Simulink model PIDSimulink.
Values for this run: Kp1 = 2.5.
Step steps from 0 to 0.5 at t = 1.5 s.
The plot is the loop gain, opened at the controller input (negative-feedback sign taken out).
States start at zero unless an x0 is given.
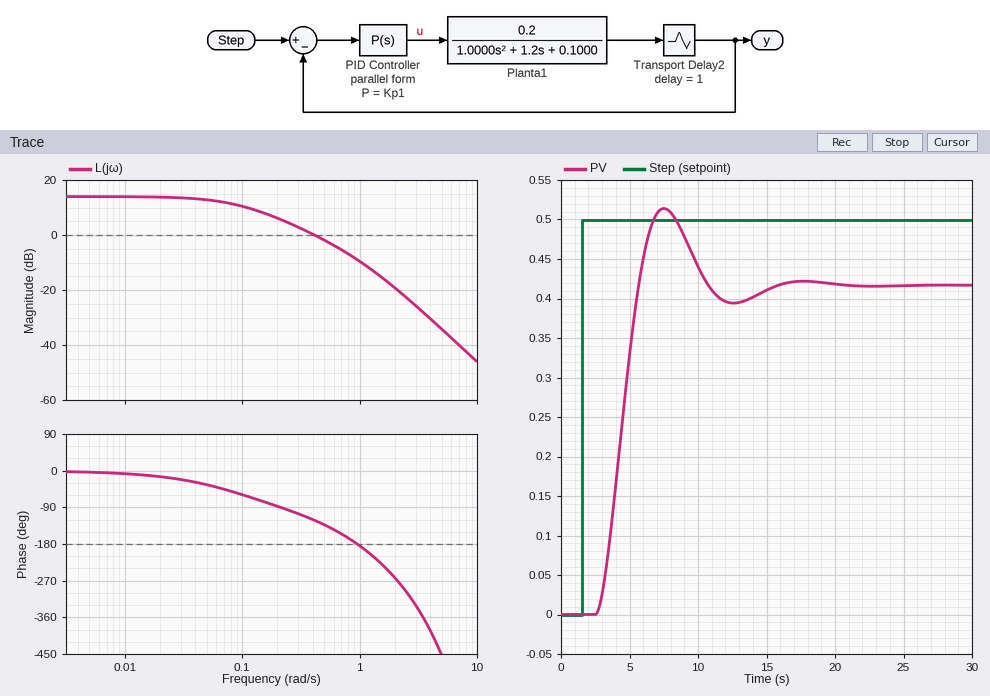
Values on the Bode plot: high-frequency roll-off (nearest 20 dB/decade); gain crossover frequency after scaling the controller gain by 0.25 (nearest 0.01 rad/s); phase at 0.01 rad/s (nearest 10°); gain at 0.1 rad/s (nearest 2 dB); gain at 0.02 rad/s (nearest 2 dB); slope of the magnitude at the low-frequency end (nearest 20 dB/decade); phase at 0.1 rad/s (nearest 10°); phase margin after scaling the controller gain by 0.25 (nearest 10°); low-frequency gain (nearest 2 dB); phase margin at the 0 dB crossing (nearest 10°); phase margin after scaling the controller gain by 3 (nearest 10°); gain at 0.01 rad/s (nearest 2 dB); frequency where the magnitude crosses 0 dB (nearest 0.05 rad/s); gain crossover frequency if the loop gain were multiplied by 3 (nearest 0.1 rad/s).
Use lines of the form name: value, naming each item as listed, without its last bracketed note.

high-frequency roll-off: -40 dB/decade
gain crossover frequency after scaling the controller gain by 0.25: 0.07 rad/s
phase at 0.01 rad/s: -10°
gain at 0.1 rad/s: 10 dB
gain at 0.02 rad/s: 14 dB
slope of the magnitude at the low-frequency end: 0 dB/decade
phase at 0.1 rad/s: -60°
phase margin after scaling the controller gain by 0.25: 140°
low-frequency gain: 14 dB
phase margin at the 0 dB crossing: 60°
phase margin after scaling the controller gain by 3: 0°
gain at 0.01 rad/s: 14 dB
frequency where the magnitude crosses 0 dB: 0.40 rad/s
gain crossover frequency if the loop gain were multiplied by 3: 1.0 rad/s
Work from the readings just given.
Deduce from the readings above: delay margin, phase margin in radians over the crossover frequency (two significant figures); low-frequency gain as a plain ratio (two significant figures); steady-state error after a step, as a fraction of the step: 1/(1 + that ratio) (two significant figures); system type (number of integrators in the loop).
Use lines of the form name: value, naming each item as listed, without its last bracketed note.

delay margin, phase margin in radians over the crossover frequency: 2.6 s
low-frequency gain as a plain ratio: 5.0
steady-state error after a step, as a fraction of the step: 1/(1 + that ratio): 0.17
system type: 0
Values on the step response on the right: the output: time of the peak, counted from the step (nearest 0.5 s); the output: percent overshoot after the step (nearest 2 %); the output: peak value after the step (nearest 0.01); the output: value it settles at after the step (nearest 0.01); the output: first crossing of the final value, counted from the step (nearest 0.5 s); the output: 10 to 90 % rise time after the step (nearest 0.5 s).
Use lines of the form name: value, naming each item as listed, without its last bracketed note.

the output: time of the peak, counted from the step: 6.0 s
the output: percent overshoot after the step: 24 %
the output: peak value after the step: 0.51
the output: value it settles at after the step: 0.42
the output: first crossing of the final value, counted from the step: 4.0 s
the output: 10 to 90 % rise time after the step: 2.0 s
